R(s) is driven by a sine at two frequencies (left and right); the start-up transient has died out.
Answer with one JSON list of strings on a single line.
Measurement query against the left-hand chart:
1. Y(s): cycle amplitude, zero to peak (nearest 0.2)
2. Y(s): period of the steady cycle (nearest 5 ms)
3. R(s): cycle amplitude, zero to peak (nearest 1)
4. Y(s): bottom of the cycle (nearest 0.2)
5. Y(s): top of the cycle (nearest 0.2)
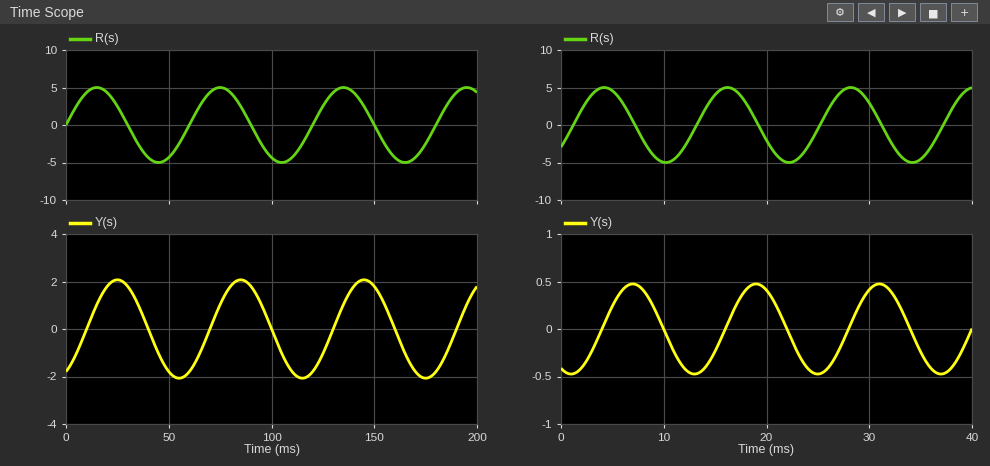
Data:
["2.0", "60 ms", "5", "-2.0", "2.0"]
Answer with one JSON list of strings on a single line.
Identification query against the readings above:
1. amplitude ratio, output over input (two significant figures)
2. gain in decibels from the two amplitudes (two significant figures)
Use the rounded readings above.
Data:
["0.40", "-8.0 dB"]
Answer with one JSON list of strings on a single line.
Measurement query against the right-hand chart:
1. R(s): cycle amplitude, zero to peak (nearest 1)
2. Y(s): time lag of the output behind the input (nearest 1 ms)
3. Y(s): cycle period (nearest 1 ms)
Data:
["5", "3 ms", "12 ms"]
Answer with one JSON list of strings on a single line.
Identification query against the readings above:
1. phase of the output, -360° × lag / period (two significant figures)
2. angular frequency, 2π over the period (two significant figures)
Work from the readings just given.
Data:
["-90°", "0.52 rad/ms"]
